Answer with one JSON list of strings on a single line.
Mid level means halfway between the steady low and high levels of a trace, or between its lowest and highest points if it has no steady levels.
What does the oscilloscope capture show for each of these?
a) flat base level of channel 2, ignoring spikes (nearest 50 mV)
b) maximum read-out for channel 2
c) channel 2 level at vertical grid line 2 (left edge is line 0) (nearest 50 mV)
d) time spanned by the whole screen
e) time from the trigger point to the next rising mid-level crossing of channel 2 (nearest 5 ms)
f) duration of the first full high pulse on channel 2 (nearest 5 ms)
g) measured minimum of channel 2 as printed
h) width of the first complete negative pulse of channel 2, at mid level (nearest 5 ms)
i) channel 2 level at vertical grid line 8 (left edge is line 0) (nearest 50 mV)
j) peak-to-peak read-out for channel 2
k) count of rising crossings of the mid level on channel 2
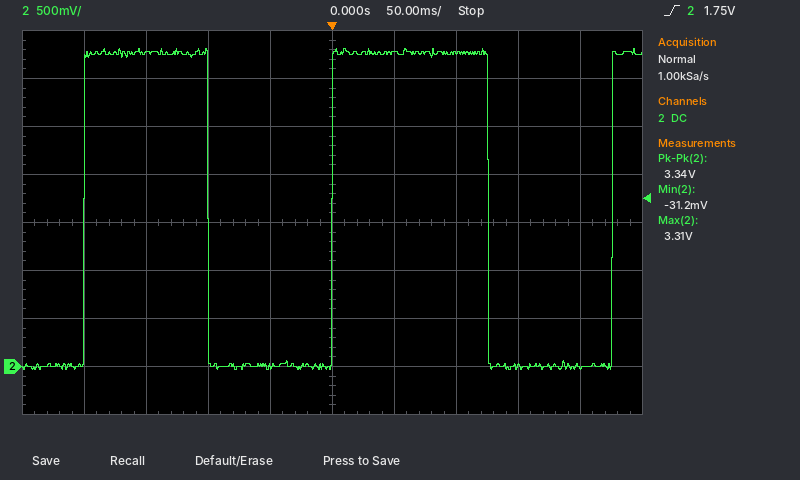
["0 mV", "3.31 V", "3.25 V", "500 ms", "225 ms", "100 ms", "-31.2 mV", "100 ms", "0 mV", "3.34 V", "3"]
